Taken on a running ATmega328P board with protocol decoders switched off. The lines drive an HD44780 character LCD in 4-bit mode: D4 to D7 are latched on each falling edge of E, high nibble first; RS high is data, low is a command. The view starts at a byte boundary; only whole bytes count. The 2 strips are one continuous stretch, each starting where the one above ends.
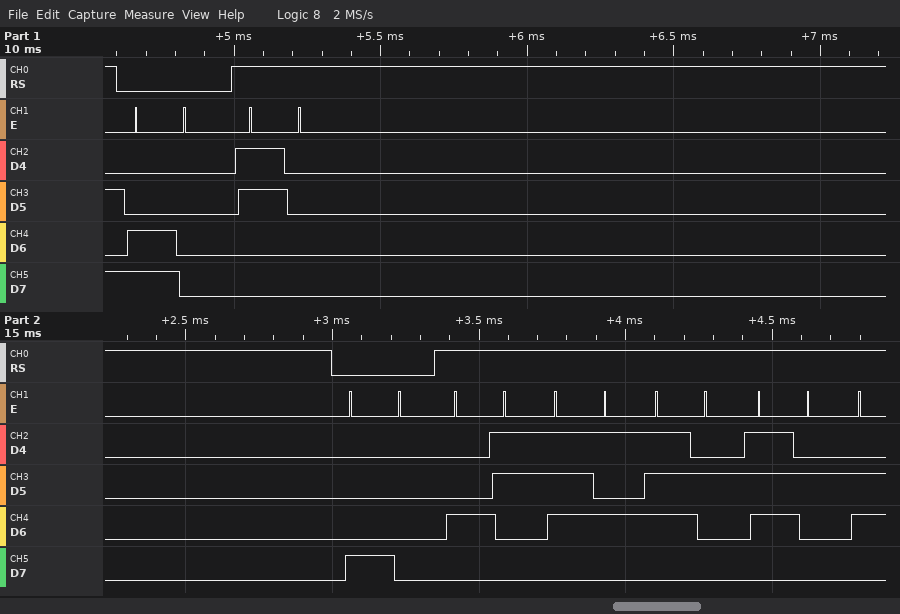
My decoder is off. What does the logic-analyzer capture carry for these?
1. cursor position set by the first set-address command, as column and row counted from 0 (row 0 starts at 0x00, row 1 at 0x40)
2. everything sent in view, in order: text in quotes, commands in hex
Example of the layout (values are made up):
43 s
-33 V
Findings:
column 0, row 1
0xC0 "0" 0x80 "Curr"
